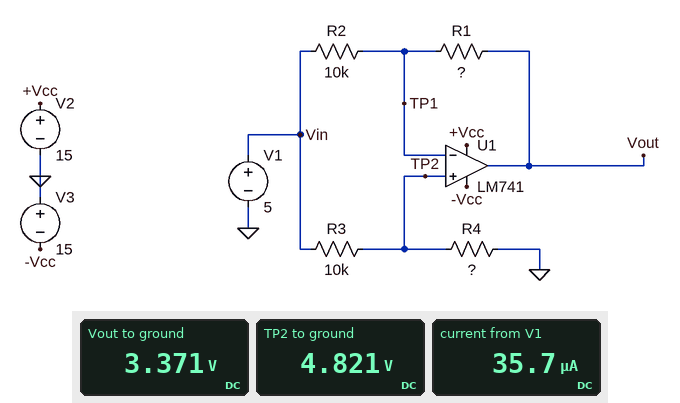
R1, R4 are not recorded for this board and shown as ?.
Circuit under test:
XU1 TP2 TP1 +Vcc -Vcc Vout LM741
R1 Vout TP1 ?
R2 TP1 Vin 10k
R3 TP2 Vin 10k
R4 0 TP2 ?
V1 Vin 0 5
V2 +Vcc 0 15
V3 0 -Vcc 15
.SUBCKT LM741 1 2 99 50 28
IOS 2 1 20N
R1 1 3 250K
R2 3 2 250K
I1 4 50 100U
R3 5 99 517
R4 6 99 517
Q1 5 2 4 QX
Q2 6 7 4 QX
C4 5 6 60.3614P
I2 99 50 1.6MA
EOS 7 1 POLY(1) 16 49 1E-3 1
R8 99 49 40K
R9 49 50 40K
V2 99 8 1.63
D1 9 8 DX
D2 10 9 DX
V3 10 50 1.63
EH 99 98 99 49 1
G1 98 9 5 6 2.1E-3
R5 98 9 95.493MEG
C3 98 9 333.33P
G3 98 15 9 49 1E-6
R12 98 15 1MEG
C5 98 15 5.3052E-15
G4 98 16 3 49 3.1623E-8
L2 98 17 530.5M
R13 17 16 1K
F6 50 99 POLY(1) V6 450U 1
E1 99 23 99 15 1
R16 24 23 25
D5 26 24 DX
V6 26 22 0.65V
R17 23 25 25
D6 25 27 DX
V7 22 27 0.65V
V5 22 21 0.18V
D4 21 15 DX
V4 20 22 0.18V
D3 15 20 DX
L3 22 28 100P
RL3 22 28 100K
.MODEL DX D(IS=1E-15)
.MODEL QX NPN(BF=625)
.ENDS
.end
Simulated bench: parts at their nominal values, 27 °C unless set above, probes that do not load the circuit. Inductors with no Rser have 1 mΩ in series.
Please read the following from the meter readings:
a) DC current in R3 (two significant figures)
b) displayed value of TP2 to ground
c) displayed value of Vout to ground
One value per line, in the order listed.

18 µA
4.821 V
3.371 V
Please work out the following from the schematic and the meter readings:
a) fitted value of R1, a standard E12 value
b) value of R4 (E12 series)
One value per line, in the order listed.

82 kΩ
270 kΩ
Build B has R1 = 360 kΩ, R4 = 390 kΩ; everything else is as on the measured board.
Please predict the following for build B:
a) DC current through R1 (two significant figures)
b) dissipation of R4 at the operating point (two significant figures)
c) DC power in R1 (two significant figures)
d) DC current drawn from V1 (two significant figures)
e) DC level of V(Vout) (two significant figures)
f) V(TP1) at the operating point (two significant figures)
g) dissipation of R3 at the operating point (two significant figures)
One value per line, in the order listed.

12 µA
61 µW
55 µW
25 µA
430 mV
4.9 V
1.6 µW
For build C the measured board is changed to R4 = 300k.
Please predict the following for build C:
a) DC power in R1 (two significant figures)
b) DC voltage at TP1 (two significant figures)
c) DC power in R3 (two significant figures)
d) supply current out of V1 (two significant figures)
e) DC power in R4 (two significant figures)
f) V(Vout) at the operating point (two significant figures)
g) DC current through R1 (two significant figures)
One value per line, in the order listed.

21 µW
4.8 V
2.6 µW
32 µA
78 µW
3.5 V
16 µA
